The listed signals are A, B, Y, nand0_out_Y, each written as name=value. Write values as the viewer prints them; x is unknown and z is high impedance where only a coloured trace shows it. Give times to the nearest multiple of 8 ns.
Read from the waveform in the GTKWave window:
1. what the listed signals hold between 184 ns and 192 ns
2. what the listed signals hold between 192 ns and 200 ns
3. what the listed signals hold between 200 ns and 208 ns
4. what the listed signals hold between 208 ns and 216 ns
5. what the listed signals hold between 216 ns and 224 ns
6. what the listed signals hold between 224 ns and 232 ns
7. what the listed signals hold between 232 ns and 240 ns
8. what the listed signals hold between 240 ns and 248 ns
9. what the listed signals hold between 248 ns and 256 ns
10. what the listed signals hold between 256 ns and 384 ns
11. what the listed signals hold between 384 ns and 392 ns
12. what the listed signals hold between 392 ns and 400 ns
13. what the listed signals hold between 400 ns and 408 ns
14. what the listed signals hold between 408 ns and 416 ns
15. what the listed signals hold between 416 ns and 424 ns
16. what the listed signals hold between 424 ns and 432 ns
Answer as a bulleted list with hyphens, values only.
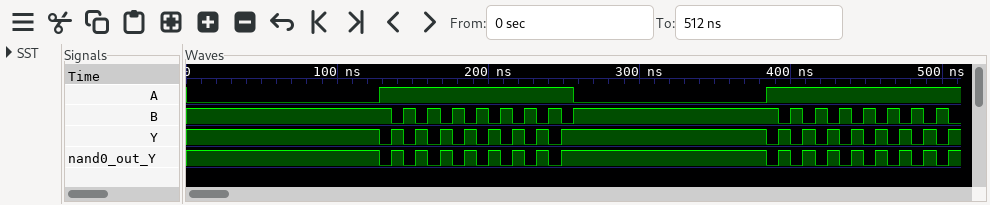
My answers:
- A=1, B=0, Y=1, nand0_out_Y=1
- A=1, B=1, Y=0, nand0_out_Y=0
- A=1, B=0, Y=1, nand0_out_Y=1
- A=1, B=1, Y=0, nand0_out_Y=0
- A=1, B=0, Y=1, nand0_out_Y=1
- A=1, B=1, Y=0, nand0_out_Y=0
- A=1, B=0, Y=1, nand0_out_Y=1
- A=1, B=1, Y=0, nand0_out_Y=0
- A=1, B=0, Y=1, nand0_out_Y=1
- A=0, B=1, Y=1, nand0_out_Y=1
- A=1, B=1, Y=0, nand0_out_Y=0
- A=1, B=0, Y=1, nand0_out_Y=1
- A=1, B=1, Y=0, nand0_out_Y=0
- A=1, B=0, Y=1, nand0_out_Y=1
- A=1, B=1, Y=0, nand0_out_Y=0
- A=1, B=0, Y=1, nand0_out_Y=1
